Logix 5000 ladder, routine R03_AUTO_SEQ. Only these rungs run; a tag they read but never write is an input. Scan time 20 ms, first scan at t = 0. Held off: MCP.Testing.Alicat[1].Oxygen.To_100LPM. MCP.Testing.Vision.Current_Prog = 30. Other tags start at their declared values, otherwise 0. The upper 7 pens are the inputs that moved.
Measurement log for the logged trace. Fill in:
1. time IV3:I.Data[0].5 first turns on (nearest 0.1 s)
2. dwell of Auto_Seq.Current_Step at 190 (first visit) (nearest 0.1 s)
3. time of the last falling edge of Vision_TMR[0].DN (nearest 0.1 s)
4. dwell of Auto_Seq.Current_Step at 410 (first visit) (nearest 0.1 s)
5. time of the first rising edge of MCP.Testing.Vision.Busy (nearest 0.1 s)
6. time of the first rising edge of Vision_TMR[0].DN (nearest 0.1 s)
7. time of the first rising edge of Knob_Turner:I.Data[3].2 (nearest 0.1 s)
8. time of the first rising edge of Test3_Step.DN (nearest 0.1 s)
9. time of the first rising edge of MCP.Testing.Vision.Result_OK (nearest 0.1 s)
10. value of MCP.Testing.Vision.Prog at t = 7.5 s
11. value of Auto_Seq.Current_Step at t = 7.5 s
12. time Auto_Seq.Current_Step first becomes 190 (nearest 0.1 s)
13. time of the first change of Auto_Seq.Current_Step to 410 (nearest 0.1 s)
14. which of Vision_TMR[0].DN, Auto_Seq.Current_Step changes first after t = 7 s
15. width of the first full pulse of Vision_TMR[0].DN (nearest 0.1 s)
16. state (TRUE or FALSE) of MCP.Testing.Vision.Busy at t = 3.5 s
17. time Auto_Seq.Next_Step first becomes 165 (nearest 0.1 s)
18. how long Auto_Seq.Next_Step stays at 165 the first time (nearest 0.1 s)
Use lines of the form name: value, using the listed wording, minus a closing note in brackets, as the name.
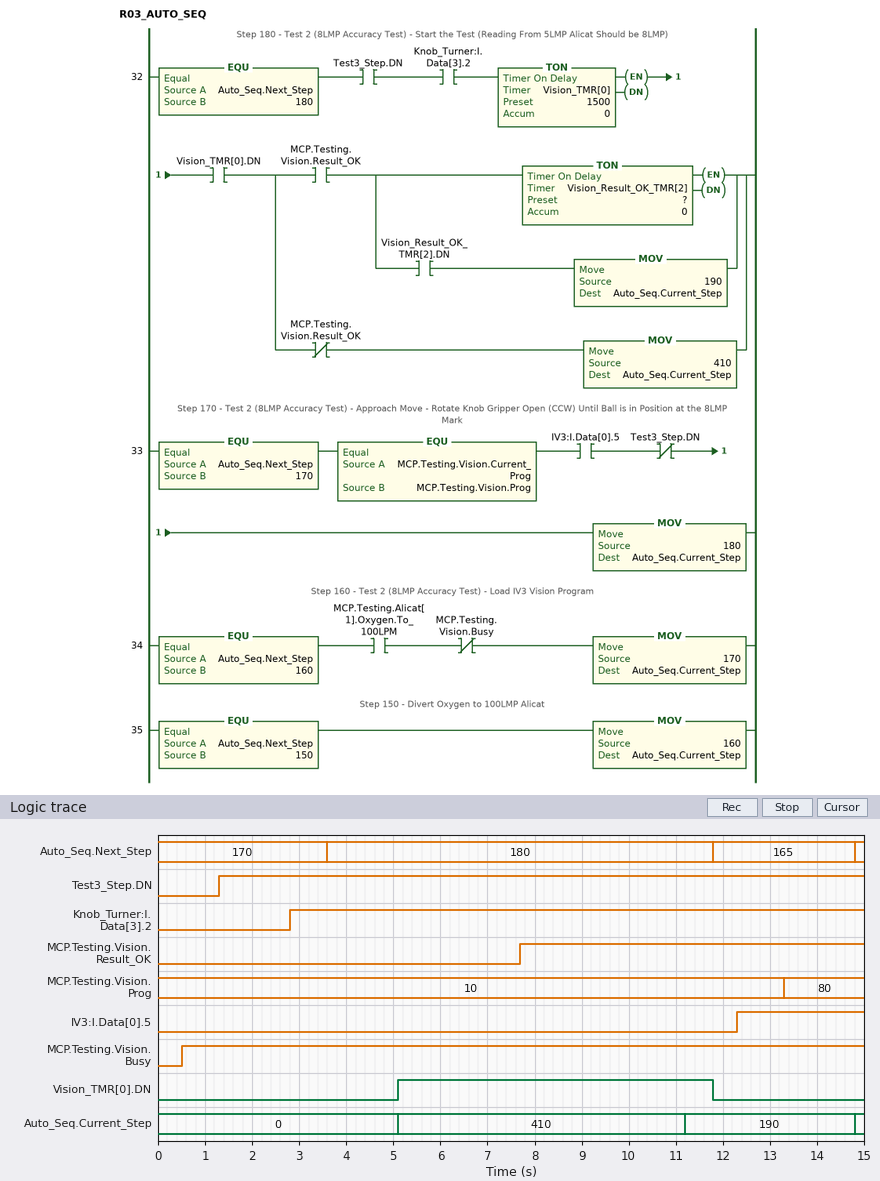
time IV3:I.Data[0].5 first turns on: 12.3 s
dwell of Auto_Seq.Current_Step at 190 (first visit): 3.6 s
time of the last falling edge of Vision_TMR[0].DN: 11.8 s
dwell of Auto_Seq.Current_Step at 410 (first visit): 6.1 s
time of the first rising edge of MCP.Testing.Vision.Busy: 0.5 s
time of the first rising edge of Vision_TMR[0].DN: 5.1 s
time of the first rising edge of Knob_Turner:I.Data[3].2: 2.8 s
time of the first rising edge of Test3_Step.DN: 1.3 s
time of the first rising edge of MCP.Testing.Vision.Result_OK: 7.7 s
value of MCP.Testing.Vision.Prog at t = 7.5 s: 10
value of Auto_Seq.Current_Step at t = 7.5 s: 410
time Auto_Seq.Current_Step first becomes 190: 11.2 s
time of the first change of Auto_Seq.Current_Step to 410: 5.1 s
which of Vision_TMR[0].DN, Auto_Seq.Current_Step changes first after t = 7 s: Auto_Seq.Current_Step
width of the first full pulse of Vision_TMR[0].DN: 6.7 s
state (TRUE or FALSE) of MCP.Testing.Vision.Busy at t = 3.5 s: TRUE
time Auto_Seq.Next_Step first becomes 165: 11.8 s
how long Auto_Seq.Next_Step stays at 165 the first time: 3.0 s
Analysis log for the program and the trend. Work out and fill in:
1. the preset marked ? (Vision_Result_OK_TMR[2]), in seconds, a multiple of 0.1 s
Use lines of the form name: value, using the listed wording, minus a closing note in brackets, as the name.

the preset marked ? (Vision_Result_OK_TMR[2]), in seconds, a multiple of 0.1 s: 3.5 s
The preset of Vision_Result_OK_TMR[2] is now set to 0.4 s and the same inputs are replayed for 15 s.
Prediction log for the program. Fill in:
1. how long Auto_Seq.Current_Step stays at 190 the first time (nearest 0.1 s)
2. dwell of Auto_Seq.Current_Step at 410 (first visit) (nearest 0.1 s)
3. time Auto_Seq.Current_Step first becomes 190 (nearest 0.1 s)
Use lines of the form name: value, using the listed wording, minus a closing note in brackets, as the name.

how long Auto_Seq.Current_Step stays at 190 the first time: 6.7 s
dwell of Auto_Seq.Current_Step at 410 (first visit): 3.0 s
time Auto_Seq.Current_Step first becomes 190: 8.1 s
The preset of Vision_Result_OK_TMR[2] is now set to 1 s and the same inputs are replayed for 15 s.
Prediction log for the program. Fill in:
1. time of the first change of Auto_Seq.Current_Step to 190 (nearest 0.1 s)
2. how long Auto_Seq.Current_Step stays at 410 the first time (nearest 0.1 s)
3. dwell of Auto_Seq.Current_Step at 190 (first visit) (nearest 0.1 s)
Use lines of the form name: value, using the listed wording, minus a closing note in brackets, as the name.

time of the first change of Auto_Seq.Current_Step to 190: 8.7 s
how long Auto_Seq.Current_Step stays at 410 the first time: 3.6 s
dwell of Auto_Seq.Current_Step at 190 (first visit): 6.1 s
